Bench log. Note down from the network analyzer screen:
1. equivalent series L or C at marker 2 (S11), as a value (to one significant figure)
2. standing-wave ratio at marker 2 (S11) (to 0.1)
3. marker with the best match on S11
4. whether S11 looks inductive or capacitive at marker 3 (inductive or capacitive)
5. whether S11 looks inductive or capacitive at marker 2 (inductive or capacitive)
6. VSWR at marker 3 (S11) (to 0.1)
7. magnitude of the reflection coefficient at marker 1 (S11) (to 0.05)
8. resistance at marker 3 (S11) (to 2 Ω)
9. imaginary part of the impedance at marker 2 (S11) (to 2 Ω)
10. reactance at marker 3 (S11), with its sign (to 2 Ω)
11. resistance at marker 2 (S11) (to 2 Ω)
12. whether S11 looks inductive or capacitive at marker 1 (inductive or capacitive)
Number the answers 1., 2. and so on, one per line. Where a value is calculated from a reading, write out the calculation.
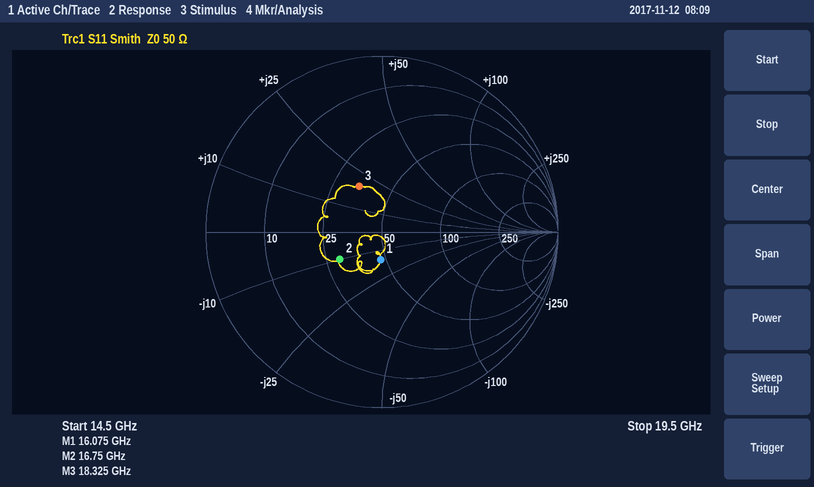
1. C = 1/(2π × 16.75 GHz × 10 Ω) ≈ 1.0 pF
2. 1.8
3. marker 1
4. inductive
5. capacitive
6. 1.8
7. 0.15
8. 34 Ω
9. -10 Ω
10. +20 Ω
11. 30 Ω
12. capacitive
